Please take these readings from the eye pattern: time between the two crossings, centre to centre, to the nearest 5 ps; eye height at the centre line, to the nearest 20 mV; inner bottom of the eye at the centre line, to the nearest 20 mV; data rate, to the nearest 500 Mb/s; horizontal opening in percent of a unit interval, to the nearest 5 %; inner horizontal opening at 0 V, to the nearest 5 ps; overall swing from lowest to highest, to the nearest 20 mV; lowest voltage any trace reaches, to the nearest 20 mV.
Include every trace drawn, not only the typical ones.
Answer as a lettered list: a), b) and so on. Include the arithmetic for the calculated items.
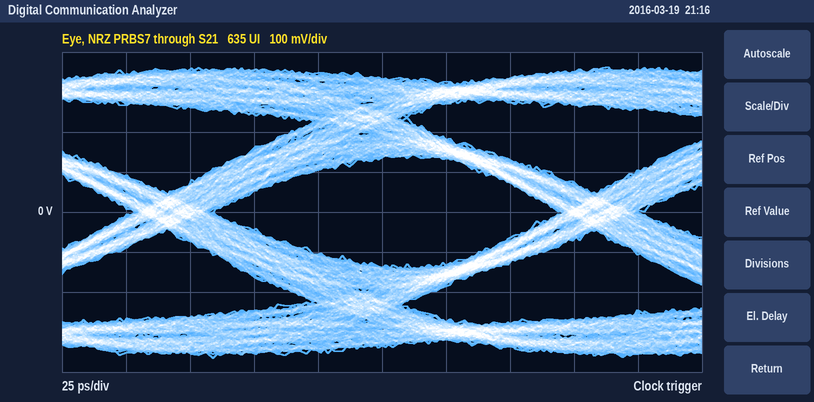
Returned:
a) 165 ps
b) 280 mV
c) -140 mV
d) 6.0 Gb/s
e) 135 ps / 165 ps ≈ 81.8 %, so 80 % to the nearest 5 %
f) 135 ps
g) 720 mV
h) -360 mV
